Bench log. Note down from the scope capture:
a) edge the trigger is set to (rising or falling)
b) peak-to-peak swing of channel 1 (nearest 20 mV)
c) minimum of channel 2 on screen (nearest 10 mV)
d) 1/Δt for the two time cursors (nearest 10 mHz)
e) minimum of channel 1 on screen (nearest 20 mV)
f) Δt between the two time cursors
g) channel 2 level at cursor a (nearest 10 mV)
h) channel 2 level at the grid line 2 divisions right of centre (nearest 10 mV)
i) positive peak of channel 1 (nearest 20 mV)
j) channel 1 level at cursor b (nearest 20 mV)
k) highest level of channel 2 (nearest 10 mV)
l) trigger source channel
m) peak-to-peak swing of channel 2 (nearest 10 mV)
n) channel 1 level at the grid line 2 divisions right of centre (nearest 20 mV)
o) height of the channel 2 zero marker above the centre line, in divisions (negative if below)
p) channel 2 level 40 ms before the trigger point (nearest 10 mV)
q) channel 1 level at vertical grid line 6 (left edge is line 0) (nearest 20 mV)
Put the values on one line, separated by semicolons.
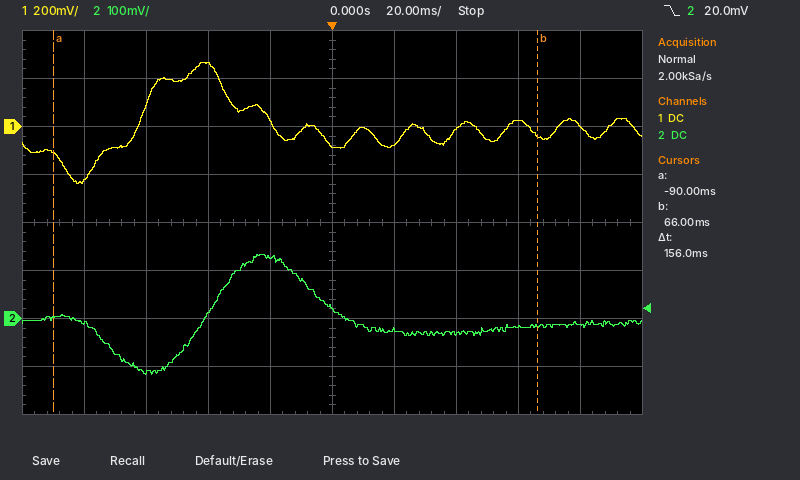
falling; 500 mV; -120 mV; 6.41 Hz; -240 mV; 156 ms; 0 mV; -30 mV; 260 mV; -40 mV; 130 mV; channel 2; 250 mV; -20 mV; -2.0 div; 10 mV; -80 mV
